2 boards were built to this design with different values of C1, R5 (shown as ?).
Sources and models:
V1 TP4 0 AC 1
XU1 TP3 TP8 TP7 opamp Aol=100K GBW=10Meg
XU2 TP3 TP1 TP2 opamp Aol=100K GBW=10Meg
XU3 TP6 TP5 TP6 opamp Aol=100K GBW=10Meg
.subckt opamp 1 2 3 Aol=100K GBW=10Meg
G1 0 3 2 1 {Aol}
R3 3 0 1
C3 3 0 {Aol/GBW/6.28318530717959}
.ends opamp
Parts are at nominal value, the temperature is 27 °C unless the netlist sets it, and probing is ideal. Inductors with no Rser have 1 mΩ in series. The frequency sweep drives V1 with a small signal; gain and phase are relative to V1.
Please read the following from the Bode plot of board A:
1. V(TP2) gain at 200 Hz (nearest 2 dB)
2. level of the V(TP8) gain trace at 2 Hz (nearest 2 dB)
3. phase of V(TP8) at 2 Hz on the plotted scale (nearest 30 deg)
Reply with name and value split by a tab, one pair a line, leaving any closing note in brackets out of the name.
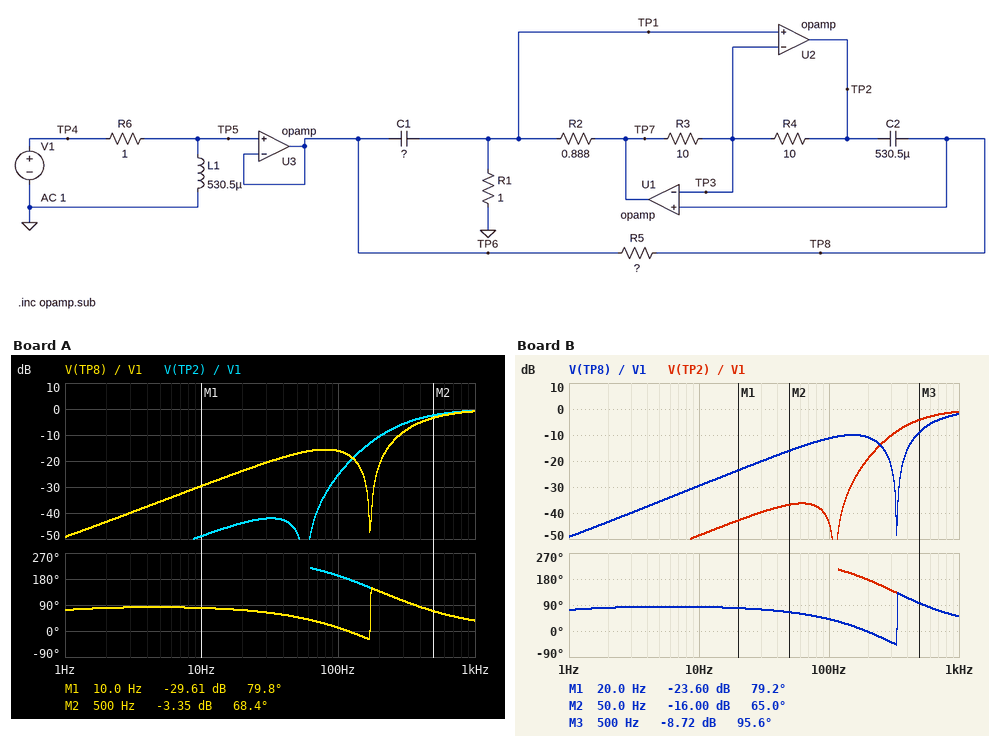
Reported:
V(TP2) gain at 200 Hz	-10 dB
level of the V(TP8) gain trace at 2 Hz	-44 dB
phase of V(TP8) at 2 Hz on the plotted scale	90 deg
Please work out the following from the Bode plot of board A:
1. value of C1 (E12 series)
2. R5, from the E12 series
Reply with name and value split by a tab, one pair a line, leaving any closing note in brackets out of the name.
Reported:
value of C1	470 µF
R5, from the E12 series	3.9 Ω
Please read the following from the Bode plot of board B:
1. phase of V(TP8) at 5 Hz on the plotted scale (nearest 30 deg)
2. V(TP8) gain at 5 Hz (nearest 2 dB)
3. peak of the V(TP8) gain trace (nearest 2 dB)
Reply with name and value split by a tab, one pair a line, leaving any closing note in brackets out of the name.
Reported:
phase of V(TP8) at 5 Hz on the plotted scale	90 deg
V(TP8) gain at 5 Hz	-36 dB
peak of the V(TP8) gain trace	-2 dB
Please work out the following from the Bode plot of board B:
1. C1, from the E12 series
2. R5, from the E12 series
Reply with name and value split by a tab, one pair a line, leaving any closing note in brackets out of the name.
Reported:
C1, from the E12 series	270 µF
R5, from the E12 series	1.8 Ω
